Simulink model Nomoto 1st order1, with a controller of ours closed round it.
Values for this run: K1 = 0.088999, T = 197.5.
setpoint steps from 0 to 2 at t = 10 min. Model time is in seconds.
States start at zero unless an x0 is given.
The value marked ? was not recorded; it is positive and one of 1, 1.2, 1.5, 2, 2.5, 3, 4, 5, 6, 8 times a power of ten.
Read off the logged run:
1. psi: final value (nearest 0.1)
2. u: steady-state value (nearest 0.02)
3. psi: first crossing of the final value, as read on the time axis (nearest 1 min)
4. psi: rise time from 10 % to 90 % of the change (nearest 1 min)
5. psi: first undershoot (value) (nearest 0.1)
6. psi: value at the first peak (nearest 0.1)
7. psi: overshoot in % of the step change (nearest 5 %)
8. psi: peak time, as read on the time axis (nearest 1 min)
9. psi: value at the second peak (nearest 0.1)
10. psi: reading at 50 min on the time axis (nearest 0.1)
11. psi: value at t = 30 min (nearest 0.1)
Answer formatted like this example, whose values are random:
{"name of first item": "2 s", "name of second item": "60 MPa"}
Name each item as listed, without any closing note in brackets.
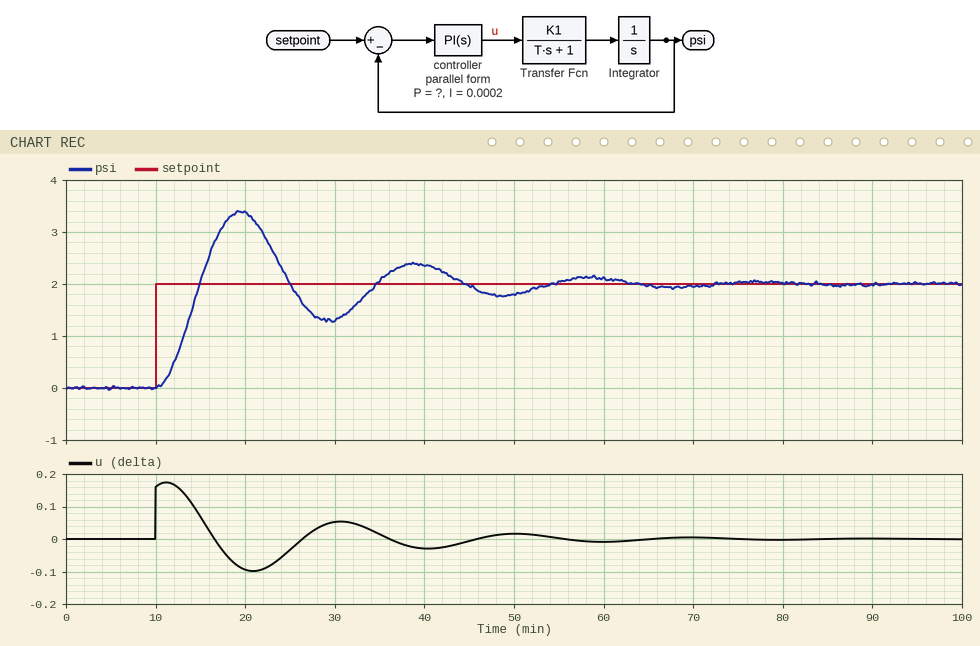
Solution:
{"psi: final value": "2.0", "u: steady-state value": "0.00", "psi: first crossing of the final value, as read on the time axis": "15 min", "psi: rise time from 10 % to 90 % of the change": "3 min", "psi: first undershoot (value)": "1.3", "psi: value at the first peak": "3.4", "psi: overshoot in % of the step change": "70 %", "psi: peak time, as read on the time axis": "19 min", "psi: value at the second peak": "2.4", "psi: reading at 50 min on the time axis": "1.8", "psi: value at t = 30 min": "1.3"}
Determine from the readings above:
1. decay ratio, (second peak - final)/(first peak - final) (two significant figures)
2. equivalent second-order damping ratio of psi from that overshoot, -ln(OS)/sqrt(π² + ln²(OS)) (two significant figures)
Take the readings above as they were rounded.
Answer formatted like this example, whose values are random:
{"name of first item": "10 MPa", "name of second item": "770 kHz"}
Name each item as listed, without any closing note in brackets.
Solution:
{"decay ratio, (second peak - final)/(first peak - final)": "0.29", "equivalent second-order damping ratio of psi from that overshoot, -ln(OS)/sqrt(π² + ln²(OS))": "0.11"}
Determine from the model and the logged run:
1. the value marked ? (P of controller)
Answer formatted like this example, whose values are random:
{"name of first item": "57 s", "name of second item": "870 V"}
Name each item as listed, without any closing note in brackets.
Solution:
{"the value marked ?": "0.08"}
